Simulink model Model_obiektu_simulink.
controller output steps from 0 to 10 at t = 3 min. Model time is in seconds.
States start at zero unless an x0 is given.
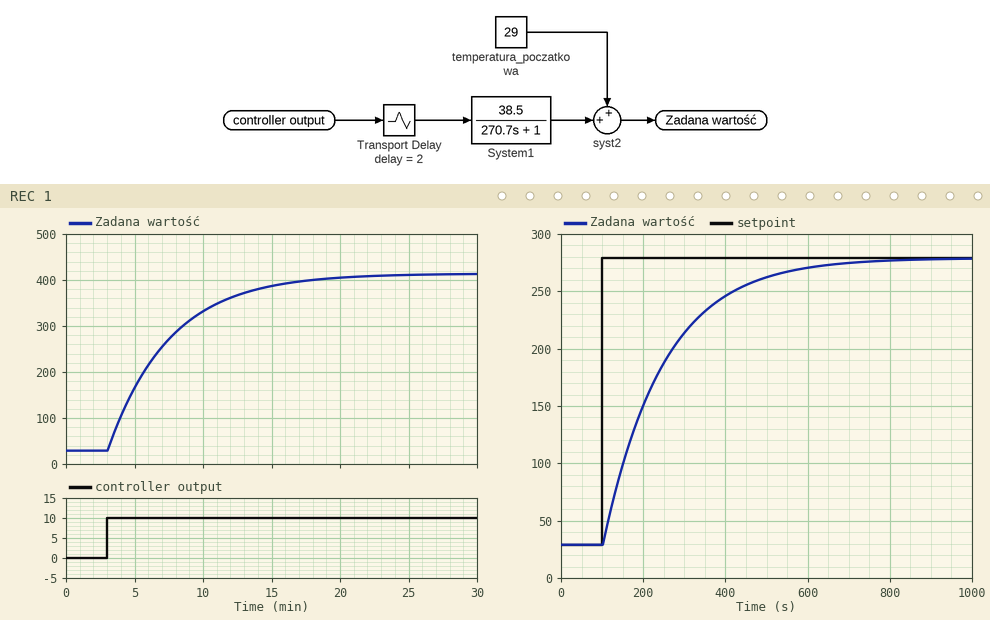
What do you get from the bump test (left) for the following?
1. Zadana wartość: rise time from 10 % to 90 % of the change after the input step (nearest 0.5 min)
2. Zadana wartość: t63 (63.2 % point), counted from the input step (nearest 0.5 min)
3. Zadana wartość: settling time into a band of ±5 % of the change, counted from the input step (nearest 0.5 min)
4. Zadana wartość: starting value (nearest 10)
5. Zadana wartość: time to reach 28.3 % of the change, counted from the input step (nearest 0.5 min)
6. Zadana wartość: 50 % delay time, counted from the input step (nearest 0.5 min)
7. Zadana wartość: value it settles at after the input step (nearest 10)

10.0 min
4.5 min
13.5 min
30
1.5 min
3.0 min
410
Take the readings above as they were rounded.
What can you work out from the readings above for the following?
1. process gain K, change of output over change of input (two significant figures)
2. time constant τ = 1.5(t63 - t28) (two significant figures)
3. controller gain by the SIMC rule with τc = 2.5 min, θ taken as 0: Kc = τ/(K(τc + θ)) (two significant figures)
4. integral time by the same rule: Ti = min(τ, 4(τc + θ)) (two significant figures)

38
4.5 min
0.047
4.5 min
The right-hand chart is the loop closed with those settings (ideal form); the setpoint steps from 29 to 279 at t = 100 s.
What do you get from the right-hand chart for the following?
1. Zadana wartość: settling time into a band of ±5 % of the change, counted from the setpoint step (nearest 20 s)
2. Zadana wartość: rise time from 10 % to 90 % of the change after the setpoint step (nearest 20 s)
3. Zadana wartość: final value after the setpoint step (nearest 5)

440 s
320 s
280
